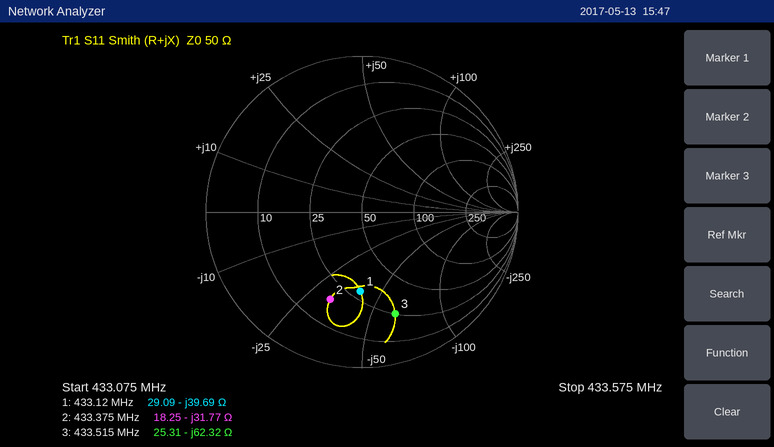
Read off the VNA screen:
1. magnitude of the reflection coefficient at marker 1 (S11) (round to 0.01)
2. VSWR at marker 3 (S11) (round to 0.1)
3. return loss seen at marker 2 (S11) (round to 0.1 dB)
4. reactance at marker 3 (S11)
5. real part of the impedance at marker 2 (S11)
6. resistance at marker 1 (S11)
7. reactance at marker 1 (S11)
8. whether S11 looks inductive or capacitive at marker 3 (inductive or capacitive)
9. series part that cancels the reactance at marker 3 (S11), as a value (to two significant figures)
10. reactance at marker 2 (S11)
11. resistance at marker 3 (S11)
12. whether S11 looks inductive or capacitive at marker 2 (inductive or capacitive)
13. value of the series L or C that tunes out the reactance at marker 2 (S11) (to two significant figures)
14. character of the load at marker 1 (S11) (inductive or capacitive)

0.51
5.4
4.5 dB
-62.32 Ω
18.25 Ω
29.09 Ω
-39.69 Ω
capacitive
23 nH
-31.77 Ω
25.31 Ω
capacitive
12 nH
capacitive
